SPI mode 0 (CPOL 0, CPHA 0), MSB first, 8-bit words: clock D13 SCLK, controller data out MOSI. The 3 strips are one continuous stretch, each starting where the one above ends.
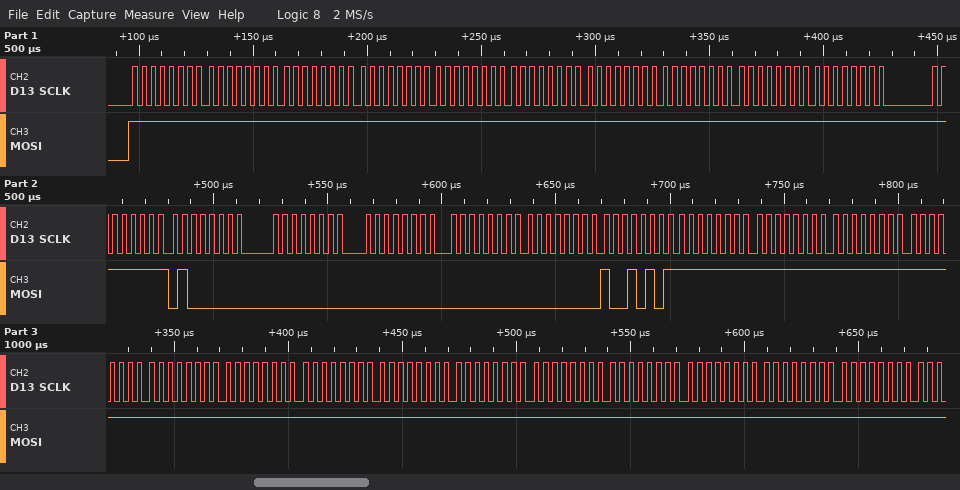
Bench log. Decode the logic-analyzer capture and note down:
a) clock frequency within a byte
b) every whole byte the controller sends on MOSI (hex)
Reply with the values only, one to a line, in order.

250 kHz
FF FF FF FF FF FF FF FF FF FF FF 40 00 00 00 00 95 FF FF FF FF FF FF FF FF FF FF FF FF FF FF
